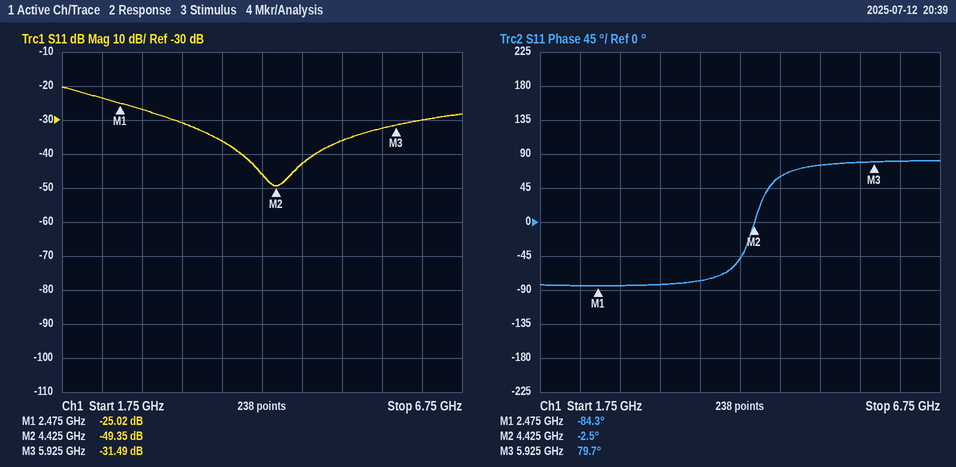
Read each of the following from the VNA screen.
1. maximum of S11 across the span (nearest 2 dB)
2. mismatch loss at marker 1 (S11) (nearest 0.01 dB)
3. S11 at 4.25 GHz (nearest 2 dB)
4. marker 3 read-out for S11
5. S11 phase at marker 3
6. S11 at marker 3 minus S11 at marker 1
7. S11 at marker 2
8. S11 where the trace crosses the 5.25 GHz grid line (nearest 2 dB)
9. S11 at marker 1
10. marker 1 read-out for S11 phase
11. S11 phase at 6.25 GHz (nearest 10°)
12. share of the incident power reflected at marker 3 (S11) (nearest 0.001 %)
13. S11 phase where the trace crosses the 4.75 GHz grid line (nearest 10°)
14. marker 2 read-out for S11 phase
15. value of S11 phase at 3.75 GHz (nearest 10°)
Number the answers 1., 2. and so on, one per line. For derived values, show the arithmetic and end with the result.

1. -20 dB
2. −10 log10(1 − 10^(-25.02/10)) ≈ 0.01 dB
3. -46 dB
4. -31.49 dB
5. 79.7°
6. -31.49 − (-25.02) = -6.47 dB
7. -49.35 dB
8. -36 dB
9. -25.02 dB
10. -84.3°
11. 80°
12. 10^(-31.49/10) ≈ 0.071 %
13. 60°
14. -2.5°
15. -80°
